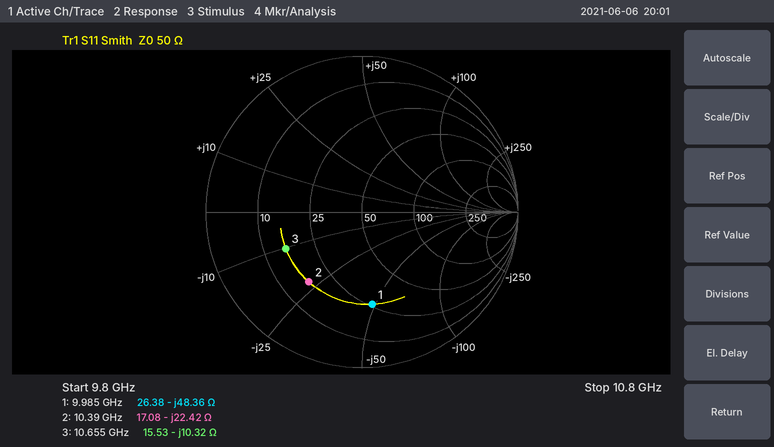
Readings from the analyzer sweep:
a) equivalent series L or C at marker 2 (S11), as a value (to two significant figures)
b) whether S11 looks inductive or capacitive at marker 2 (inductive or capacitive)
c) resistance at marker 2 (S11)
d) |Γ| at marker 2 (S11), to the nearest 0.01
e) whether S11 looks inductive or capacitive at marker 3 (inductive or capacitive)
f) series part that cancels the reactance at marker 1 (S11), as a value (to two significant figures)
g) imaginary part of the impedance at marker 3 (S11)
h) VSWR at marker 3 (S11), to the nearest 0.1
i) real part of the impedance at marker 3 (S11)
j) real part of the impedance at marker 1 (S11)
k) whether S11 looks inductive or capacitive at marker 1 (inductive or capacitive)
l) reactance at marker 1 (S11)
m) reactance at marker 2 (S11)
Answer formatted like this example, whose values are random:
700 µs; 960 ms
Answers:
680 fF; capacitive; 17.08 Ω; 0.56; capacitive; 770 pH; -10.32 Ω; 3.4; 15.53 Ω; 26.38 Ω; capacitive; -48.36 Ω; -22.42 Ω
